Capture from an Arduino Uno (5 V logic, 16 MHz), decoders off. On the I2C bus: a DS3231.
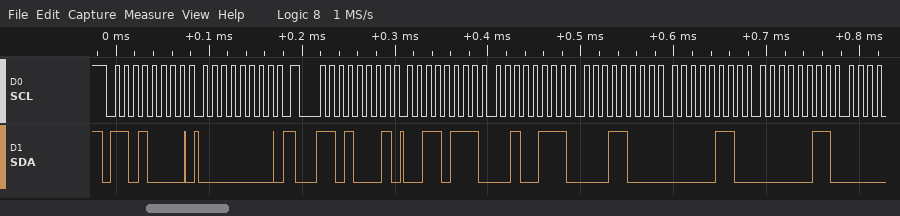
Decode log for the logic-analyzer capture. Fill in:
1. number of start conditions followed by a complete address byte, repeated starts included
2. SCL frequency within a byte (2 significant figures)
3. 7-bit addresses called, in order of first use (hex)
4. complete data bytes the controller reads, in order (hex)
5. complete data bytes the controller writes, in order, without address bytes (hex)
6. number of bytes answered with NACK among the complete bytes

2
100 kHz
0x68
37 27 18 06 03
00
0
